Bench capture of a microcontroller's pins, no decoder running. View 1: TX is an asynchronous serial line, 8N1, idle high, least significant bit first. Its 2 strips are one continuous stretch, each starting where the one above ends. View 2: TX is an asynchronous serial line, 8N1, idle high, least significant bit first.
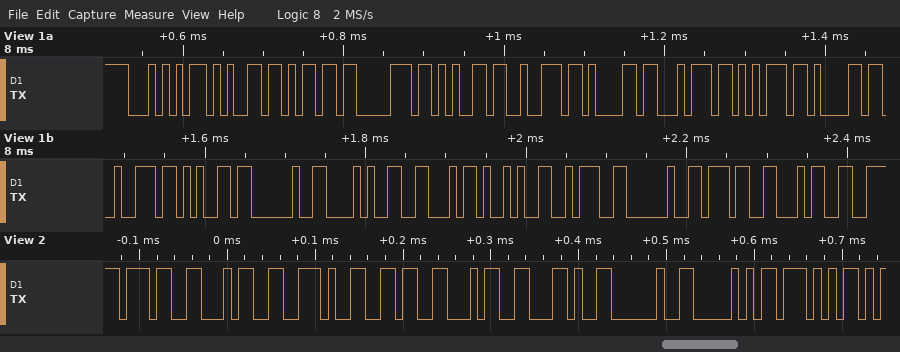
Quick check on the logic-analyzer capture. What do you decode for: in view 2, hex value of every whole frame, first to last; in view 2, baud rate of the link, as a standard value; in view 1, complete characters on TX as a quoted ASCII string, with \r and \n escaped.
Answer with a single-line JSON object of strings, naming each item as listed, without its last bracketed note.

{"in view 2, hex value of every whole frame, first to last": "0x37 0x34 0x2E 0x36 0x34 0x2C 0x20 0x50 0x57", "in view 2, baud rate of the link, as a standard value": "115200 baud", "in view 1, complete characters on TX as a quoted ASCII string, with \\r and \\n escaped": "\"Temperatuare (F): 74\""}
